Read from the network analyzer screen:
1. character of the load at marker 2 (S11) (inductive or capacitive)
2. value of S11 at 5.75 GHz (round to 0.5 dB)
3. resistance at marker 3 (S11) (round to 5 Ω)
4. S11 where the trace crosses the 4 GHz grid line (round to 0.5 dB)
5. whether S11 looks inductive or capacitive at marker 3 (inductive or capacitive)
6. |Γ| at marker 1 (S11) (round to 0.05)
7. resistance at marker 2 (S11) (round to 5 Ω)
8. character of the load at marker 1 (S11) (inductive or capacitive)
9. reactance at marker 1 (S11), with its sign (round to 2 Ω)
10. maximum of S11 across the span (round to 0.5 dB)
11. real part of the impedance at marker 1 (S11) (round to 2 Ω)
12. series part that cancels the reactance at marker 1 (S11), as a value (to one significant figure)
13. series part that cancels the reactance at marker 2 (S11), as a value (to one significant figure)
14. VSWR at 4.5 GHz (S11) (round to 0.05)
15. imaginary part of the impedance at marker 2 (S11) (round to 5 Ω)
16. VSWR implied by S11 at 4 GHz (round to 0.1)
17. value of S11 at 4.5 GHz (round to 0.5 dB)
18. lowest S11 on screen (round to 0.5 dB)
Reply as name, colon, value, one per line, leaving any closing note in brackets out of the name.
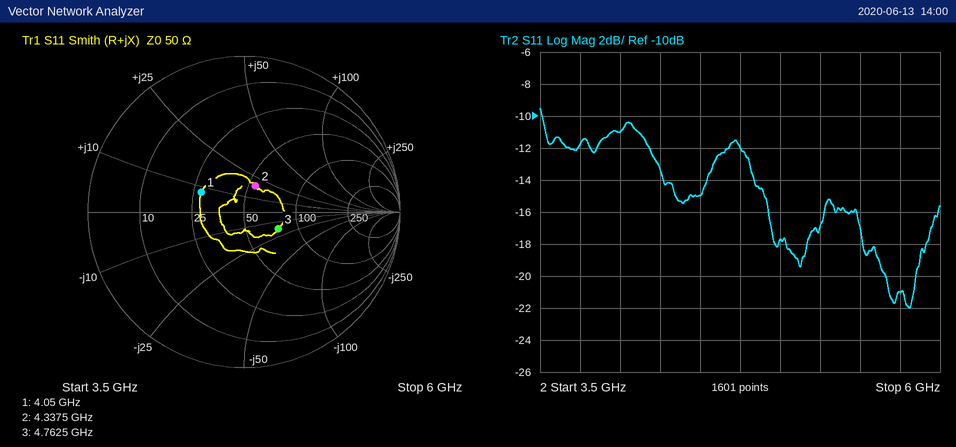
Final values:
character of the load at marker 2 (S11): inductive
value of S11 at 5.75 GHz: -21.0 dB
resistance at marker 3 (S11): 75 Ω
S11 where the trace crosses the 4 GHz grid line: -11.0 dB
whether S11 looks inductive or capacitive at marker 3: capacitive
|Γ| at marker 1 (S11): 0.30
resistance at marker 2 (S11): 55 Ω
character of the load at marker 1 (S11): inductive
reactance at marker 1 (S11), with its sign: +8 Ω
maximum of S11 across the span: -9.5 dB
real part of the impedance at marker 1 (S11): 28 Ω
series part that cancels the reactance at marker 1 (S11), as a value: 5 pF
series part that cancels the reactance at marker 2 (S11), as a value: 2 pF
VSWR at 4.5 GHz (S11): 1.45
imaginary part of the impedance at marker 2 (S11): +20 Ω
VSWR implied by S11 at 4 GHz: 1.8
value of S11 at 4.5 GHz: -15.0 dB
lowest S11 on screen: -22.0 dB
